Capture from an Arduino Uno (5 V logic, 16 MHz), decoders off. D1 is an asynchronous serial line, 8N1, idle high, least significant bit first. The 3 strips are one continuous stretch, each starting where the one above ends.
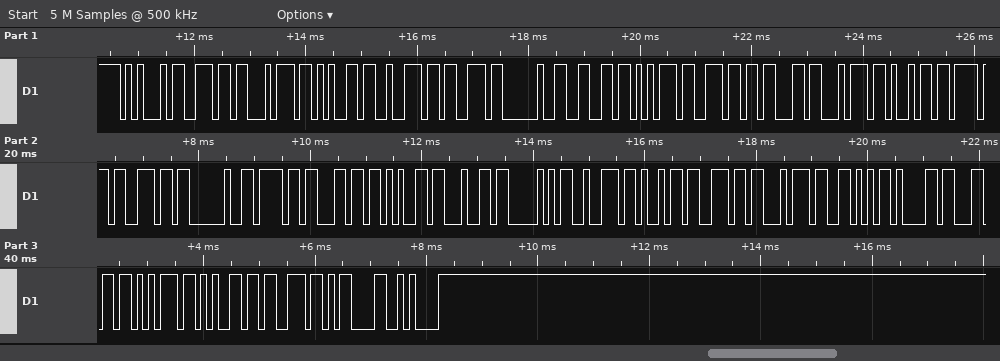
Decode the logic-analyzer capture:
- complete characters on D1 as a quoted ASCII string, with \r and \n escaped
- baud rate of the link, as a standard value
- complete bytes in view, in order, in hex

"Enters function oledPrintValues\r\n"
9600 baud
45 6E 74 65 72 73 20 66 75 6E 63 74 69 6F 6E 20 6F 6C 65 64 50 72 69 6E 74 56 61 6C 75 65 73 0D 0A
